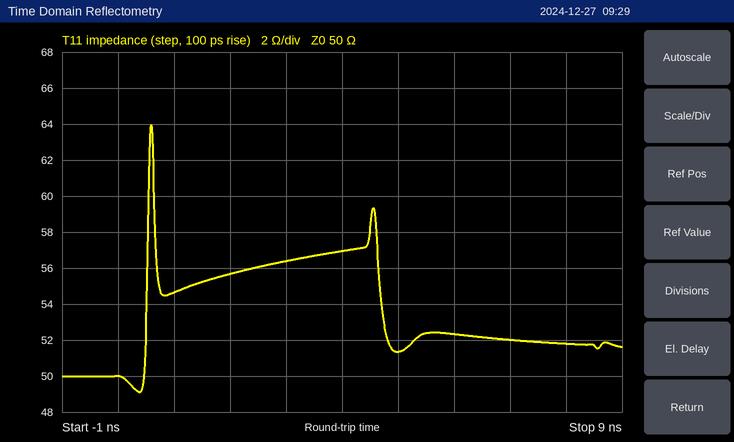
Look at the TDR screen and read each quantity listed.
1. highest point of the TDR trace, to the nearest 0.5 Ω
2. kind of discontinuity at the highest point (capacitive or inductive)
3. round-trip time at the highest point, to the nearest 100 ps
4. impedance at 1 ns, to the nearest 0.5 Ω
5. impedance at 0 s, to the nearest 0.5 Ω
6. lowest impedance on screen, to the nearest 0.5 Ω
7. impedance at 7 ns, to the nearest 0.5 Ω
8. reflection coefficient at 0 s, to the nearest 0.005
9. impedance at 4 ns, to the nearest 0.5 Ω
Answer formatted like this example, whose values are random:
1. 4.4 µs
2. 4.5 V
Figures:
1. 64.0 Ω
2. inductive
3. 600 ps
4. 54.5 Ω
5. 50.0 Ω
6. 49.0 Ω
7. 52.0 Ω
8. 0.000
9. 57.0 Ω
